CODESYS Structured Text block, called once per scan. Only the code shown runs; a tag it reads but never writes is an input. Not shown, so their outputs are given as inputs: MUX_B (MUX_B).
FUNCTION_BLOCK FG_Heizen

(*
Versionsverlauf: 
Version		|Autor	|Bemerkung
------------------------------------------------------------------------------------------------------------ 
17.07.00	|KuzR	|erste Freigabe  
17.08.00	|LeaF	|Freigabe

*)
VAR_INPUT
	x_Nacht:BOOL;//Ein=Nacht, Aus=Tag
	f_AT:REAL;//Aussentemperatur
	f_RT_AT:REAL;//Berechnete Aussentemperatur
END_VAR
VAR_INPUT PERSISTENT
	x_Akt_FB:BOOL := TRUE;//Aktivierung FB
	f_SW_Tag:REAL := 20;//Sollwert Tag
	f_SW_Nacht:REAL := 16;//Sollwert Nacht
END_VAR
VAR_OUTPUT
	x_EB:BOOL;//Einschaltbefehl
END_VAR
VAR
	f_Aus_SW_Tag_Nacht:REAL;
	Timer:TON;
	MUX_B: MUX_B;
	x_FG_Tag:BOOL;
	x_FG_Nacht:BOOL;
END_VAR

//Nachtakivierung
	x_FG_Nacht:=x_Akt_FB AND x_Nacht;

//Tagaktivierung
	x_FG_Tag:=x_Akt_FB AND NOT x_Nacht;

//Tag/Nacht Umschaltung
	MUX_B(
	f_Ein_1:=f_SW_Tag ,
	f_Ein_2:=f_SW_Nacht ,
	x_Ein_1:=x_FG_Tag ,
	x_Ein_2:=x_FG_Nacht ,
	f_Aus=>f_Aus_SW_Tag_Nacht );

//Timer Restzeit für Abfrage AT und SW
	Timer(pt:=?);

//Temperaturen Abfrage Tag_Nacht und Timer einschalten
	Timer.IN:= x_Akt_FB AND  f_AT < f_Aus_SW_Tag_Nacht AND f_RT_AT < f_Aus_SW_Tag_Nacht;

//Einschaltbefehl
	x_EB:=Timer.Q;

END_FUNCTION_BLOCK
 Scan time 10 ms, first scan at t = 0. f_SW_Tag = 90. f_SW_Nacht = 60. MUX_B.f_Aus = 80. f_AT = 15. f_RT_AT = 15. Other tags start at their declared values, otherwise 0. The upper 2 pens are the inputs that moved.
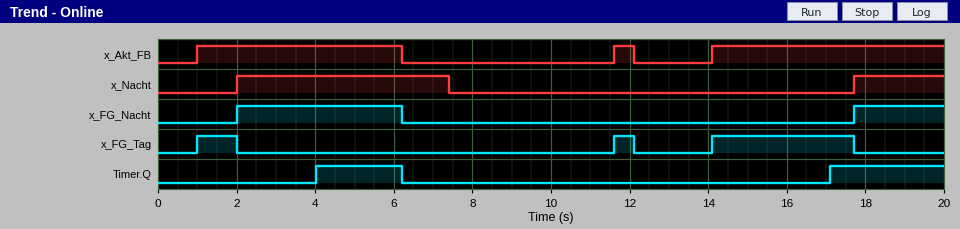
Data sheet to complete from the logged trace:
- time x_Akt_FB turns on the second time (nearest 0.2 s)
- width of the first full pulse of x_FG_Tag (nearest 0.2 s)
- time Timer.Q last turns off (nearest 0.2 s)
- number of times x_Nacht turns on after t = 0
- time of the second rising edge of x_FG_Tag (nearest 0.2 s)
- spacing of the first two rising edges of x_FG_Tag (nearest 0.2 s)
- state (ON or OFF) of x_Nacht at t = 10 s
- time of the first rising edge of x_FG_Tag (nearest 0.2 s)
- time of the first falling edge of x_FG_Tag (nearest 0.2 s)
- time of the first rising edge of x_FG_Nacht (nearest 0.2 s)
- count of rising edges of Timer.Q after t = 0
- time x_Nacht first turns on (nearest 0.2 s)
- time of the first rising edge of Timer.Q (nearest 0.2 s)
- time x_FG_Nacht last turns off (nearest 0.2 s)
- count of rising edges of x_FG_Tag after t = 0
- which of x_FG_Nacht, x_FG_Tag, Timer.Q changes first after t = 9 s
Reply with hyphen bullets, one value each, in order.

- 11.6 s
- 1.0 s
- 6.2 s
- 2
- 11.6 s
- 10.6 s
- OFF
- 1.0 s
- 2.0 s
- 2.0 s
- 2
- 2.0 s
- 4.0 s
- 6.2 s
- 3
- x_FG_Tag
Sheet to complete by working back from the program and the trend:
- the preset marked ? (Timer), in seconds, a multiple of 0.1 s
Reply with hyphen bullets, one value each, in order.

- 3.0 s
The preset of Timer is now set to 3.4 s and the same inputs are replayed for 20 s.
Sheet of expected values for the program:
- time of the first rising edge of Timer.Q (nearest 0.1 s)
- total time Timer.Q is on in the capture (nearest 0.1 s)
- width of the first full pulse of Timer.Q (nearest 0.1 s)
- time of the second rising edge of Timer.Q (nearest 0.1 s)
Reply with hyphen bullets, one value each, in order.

- 4.4 s
- 4.3 s
- 1.8 s
- 17.5 s
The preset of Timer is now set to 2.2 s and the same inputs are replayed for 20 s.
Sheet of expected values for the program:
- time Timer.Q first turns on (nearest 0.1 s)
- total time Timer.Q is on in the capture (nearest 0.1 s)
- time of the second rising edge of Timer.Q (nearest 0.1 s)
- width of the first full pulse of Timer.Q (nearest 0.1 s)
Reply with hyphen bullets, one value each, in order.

- 3.2 s
- 6.7 s
- 16.3 s
- 3.0 s
